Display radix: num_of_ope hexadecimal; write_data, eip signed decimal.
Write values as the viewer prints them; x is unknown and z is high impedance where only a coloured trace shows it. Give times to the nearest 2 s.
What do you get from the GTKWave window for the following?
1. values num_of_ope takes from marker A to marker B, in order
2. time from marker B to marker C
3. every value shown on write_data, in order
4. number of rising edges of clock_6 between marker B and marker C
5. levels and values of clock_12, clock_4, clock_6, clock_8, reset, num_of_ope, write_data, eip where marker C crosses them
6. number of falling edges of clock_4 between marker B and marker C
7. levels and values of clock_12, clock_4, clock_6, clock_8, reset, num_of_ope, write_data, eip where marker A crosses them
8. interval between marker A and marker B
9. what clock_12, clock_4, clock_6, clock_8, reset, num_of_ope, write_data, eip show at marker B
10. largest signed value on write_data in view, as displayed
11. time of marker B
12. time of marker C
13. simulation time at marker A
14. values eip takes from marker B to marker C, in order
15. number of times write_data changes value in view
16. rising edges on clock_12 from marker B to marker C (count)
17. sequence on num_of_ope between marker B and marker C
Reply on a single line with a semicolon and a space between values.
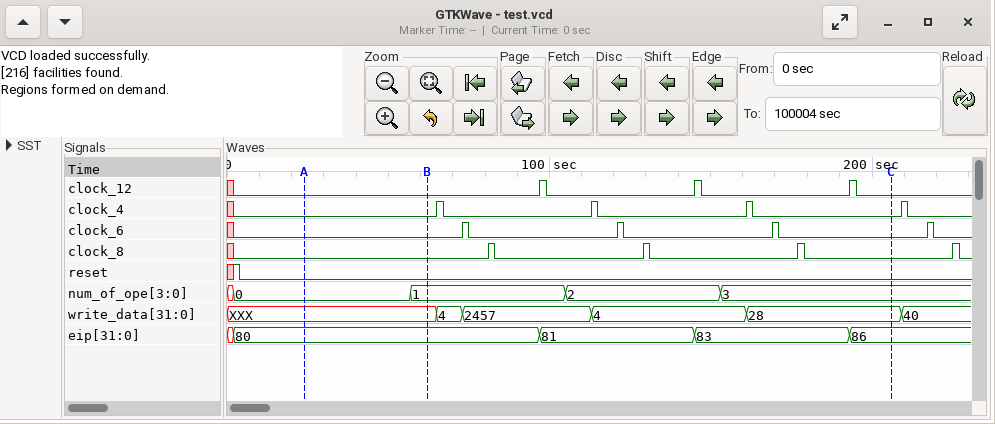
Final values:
0, 1; 144 s; XXX, 4, 2457, 4, 28, 40; 3; clock_12=0, clock_4=0, clock_6=0, clock_8=0, reset=0, num_of_ope=3, write_data=28, eip=86; 3; clock_12=0, clock_4=0, clock_6=0, clock_8=0, reset=0, num_of_ope=0, write_data=XXX, eip=80; 38 s; clock_12=0, clock_4=0, clock_6=0, clock_8=0, reset=0, num_of_ope=1, write_data=XXX, eip=80; 2457; 62 s; 206 s; 24 s; 80, 81, 83, 86; 5; 3; 1, 2, 3
